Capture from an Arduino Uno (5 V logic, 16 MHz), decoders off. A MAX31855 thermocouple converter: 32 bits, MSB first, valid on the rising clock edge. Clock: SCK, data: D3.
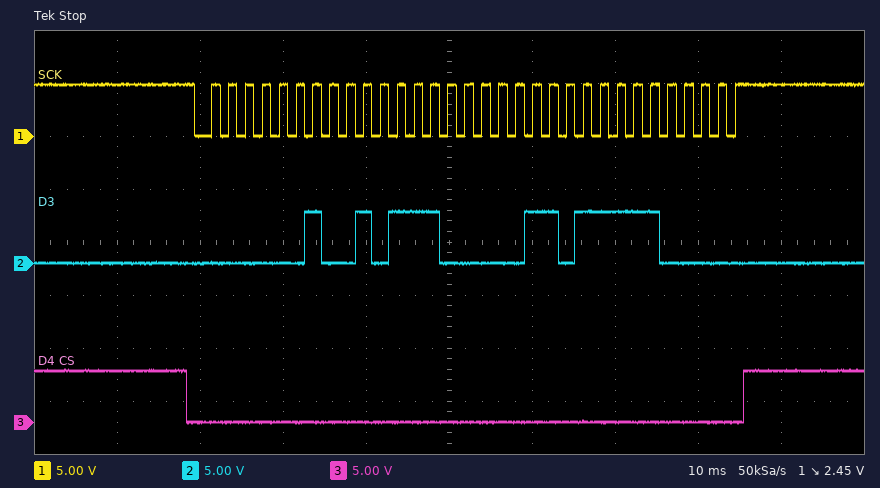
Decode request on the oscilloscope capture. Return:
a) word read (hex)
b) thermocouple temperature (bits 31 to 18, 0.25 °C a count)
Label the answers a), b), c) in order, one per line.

a) 0x025C1BE0
b) 37.75 °C
